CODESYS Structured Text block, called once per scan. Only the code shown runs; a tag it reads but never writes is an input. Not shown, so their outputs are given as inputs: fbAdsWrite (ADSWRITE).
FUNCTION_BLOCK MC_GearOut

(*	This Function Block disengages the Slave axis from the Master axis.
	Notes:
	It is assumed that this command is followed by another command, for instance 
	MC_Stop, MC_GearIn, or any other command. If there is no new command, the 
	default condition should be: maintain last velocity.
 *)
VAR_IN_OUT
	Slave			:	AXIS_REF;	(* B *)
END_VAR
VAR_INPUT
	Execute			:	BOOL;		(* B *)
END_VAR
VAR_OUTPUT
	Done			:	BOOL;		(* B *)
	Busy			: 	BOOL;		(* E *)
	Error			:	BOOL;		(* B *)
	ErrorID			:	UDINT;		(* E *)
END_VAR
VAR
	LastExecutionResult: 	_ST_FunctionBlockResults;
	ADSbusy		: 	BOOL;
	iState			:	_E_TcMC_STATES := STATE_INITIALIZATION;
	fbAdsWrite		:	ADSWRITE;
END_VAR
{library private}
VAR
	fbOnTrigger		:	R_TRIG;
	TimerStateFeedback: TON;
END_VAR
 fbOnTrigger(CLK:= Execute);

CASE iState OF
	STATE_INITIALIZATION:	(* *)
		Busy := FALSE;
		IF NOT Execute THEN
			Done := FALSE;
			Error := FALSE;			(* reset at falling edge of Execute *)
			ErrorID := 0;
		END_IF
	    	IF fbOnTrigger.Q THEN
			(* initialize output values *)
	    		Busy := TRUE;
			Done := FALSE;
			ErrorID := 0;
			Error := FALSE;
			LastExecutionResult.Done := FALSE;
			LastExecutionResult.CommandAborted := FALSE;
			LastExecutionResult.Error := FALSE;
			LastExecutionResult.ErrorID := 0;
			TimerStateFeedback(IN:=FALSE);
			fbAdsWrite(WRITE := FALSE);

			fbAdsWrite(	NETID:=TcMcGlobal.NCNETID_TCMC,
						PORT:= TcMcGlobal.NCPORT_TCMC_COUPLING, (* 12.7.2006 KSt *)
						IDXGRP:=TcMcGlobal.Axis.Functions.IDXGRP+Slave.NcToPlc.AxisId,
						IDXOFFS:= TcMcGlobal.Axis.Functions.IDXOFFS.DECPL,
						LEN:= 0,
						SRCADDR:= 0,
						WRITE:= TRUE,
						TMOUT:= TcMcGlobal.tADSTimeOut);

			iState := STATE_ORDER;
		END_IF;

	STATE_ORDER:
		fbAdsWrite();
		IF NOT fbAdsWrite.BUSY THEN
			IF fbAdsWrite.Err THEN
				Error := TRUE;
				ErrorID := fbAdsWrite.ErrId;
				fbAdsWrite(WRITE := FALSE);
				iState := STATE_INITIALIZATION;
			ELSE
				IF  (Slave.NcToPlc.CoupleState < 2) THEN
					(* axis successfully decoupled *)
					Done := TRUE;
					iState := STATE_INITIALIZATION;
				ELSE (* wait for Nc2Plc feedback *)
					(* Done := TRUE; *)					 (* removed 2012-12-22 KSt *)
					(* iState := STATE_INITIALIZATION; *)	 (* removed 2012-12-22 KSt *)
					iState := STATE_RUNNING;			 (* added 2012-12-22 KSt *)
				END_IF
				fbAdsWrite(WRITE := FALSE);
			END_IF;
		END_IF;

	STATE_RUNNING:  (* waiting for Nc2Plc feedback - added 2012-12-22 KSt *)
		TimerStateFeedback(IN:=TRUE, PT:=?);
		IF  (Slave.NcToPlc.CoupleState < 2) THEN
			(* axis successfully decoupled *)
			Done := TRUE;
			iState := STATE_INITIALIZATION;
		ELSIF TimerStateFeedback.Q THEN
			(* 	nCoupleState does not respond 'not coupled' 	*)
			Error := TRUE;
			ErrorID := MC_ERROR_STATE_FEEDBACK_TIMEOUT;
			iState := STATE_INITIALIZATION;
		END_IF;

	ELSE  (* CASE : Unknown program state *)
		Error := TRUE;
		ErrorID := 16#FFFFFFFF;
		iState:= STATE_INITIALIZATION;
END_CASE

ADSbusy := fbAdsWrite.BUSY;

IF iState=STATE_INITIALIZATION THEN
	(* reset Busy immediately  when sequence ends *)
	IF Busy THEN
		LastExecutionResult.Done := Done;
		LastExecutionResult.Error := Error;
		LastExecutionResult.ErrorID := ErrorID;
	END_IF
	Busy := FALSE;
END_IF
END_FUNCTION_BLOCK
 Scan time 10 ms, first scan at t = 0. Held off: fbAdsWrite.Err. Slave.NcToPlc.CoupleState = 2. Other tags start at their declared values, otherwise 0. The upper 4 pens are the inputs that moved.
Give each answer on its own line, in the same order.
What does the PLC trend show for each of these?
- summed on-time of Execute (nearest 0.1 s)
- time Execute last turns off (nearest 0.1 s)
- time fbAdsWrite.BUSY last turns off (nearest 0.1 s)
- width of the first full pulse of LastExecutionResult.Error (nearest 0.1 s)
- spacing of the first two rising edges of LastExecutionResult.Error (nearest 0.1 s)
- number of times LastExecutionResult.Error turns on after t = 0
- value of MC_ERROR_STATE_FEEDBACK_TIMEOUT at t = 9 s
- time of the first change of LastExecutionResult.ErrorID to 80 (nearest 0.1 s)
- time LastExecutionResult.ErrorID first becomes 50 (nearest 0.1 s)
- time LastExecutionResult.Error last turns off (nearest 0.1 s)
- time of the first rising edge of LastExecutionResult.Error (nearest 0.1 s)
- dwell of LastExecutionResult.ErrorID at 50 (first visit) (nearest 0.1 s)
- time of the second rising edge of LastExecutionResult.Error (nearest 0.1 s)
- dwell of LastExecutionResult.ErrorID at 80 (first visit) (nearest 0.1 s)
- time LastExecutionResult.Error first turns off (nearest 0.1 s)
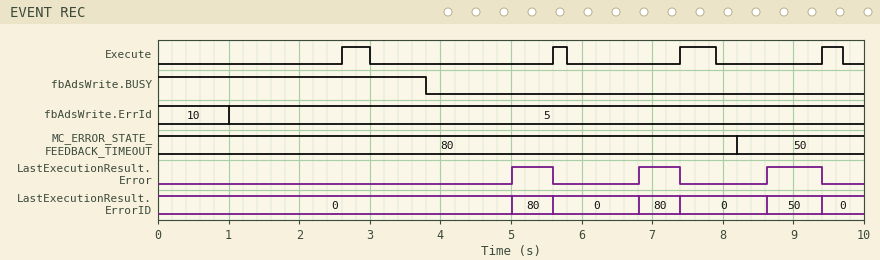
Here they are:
1.4 s
9.7 s
3.8 s
0.6 s
1.8 s
3
50
5.0 s
8.6 s
9.4 s
5.0 s
0.8 s
6.8 s
0.6 s
5.6 s
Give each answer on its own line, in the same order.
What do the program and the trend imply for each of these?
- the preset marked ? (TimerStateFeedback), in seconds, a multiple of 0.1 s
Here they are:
1.2 s
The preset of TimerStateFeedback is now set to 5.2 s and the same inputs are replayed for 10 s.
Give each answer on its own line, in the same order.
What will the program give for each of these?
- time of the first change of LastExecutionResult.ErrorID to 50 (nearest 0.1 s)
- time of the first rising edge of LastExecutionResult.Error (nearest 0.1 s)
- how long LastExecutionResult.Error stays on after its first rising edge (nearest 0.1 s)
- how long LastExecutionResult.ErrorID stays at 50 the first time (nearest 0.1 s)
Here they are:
9.0 s
9.0 s
0.4 s
0.4 s
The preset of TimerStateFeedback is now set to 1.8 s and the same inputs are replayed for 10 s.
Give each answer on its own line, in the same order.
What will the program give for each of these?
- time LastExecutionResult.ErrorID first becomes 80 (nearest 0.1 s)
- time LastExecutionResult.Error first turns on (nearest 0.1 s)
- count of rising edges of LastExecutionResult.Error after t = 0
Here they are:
5.6 s
5.6 s
2
